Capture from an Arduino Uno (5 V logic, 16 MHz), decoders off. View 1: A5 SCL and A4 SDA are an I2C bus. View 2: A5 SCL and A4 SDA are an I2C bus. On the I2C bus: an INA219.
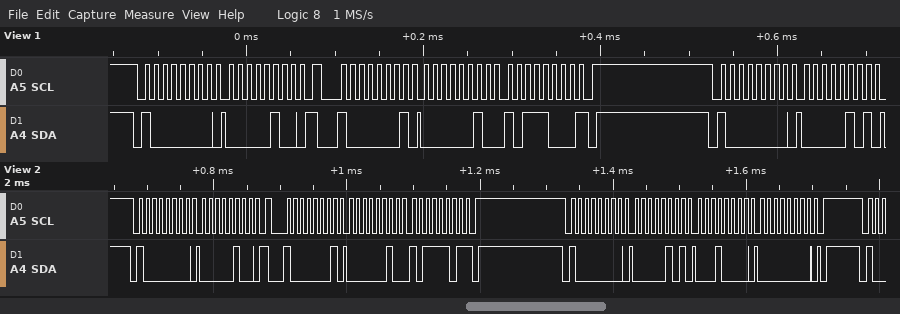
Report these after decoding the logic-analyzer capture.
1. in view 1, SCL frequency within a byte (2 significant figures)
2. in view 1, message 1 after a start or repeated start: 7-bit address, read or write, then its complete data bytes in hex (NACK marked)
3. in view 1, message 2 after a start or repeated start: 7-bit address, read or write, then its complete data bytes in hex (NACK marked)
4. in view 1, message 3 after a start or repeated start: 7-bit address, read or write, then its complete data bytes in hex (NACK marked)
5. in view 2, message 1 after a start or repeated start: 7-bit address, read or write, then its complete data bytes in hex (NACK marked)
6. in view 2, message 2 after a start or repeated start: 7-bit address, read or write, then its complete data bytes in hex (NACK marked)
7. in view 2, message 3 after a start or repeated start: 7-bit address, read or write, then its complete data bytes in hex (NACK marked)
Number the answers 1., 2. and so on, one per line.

1. 100 kHz
2. 0x40 write: 04
3. 0x40 read: 02 B8 NACK
4. 0x40 write: 05
5. 0x40 write: 04
6. 0x40 read: 02 BD NACK
7. 0x40 write: 05 10 00
